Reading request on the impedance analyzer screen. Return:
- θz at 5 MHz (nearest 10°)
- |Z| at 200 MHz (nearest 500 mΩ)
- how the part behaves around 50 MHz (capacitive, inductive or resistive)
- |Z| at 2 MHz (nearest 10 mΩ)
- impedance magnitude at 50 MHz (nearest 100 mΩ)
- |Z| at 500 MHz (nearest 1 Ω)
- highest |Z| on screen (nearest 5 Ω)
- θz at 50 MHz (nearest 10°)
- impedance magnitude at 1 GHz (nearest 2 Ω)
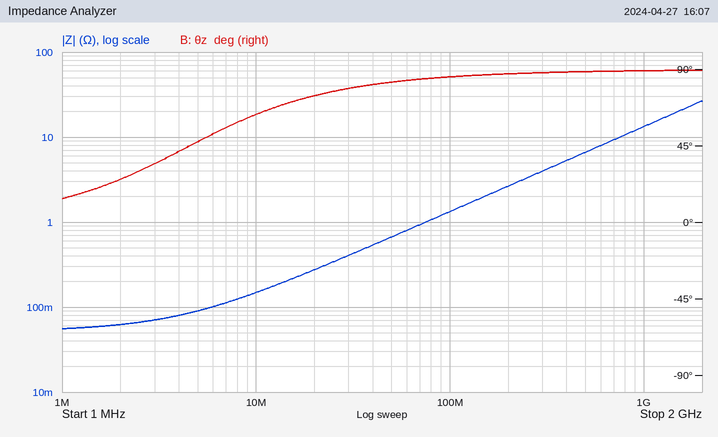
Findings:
50°
2.5 Ω
inductive
60 mΩ
700 mΩ
7 Ω
25 Ω
80°
14 Ω
